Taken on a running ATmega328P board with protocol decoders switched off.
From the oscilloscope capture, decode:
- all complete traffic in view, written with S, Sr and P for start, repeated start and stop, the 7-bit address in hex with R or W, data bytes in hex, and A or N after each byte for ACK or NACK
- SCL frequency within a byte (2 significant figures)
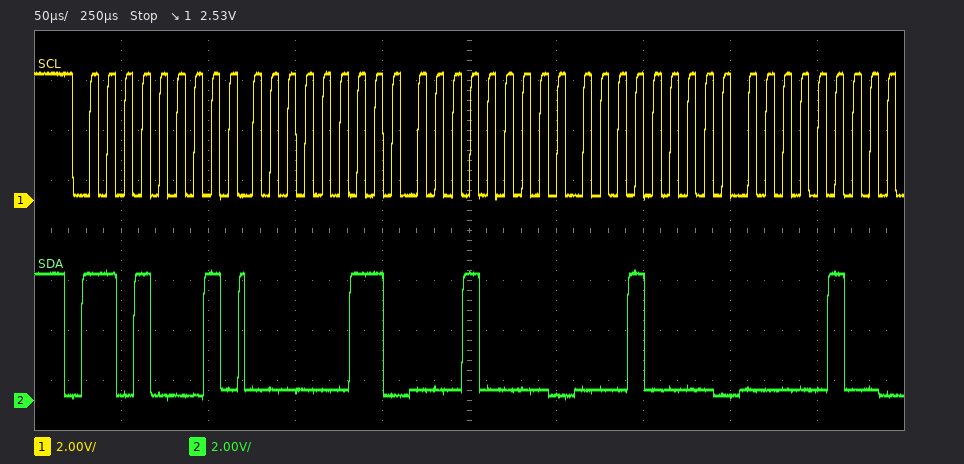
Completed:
S 68R A 03 A 10 A 10 A 04 A
100 kHz
